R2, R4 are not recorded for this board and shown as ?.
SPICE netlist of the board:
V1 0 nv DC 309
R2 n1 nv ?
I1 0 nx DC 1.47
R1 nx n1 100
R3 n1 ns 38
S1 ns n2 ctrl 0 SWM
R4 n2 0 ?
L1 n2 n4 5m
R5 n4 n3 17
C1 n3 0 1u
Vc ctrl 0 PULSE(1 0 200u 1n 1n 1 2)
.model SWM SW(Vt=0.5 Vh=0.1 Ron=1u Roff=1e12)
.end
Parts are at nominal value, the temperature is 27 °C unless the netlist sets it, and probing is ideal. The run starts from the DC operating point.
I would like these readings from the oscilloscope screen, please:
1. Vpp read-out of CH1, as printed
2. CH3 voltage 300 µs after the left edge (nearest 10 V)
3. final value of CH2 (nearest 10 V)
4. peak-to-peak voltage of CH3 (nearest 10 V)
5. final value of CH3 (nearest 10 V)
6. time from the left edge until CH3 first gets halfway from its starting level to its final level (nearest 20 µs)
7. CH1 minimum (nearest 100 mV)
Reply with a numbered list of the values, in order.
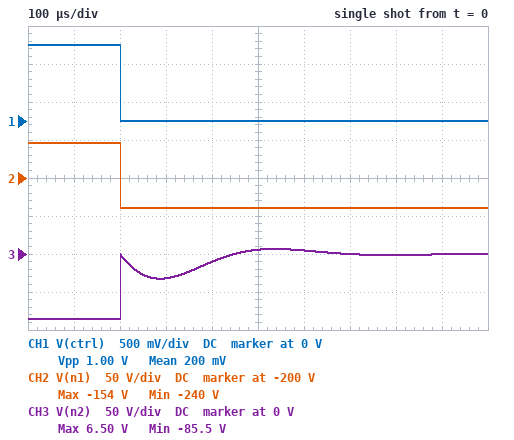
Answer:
1. 1.00 V
2. -30 V
3. -240 V
4. 90 V
5. 0 V
6. 200 µs
7. 0 V
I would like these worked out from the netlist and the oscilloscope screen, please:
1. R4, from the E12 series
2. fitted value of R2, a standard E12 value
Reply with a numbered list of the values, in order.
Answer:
1. 47 Ω
2. 47 Ω
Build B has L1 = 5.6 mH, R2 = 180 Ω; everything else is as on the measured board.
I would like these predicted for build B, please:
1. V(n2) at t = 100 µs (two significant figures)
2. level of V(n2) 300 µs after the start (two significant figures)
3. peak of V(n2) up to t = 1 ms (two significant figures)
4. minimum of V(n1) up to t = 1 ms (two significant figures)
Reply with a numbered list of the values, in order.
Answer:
1. -7.9 V
2. -2.9 V
3. 660 mV
4. -44 V
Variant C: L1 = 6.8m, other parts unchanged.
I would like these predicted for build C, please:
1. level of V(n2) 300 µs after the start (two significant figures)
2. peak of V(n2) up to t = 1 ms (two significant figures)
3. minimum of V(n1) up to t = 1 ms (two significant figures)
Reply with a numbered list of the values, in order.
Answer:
1. -30 V
2. 7.9 V
3. -240 V
